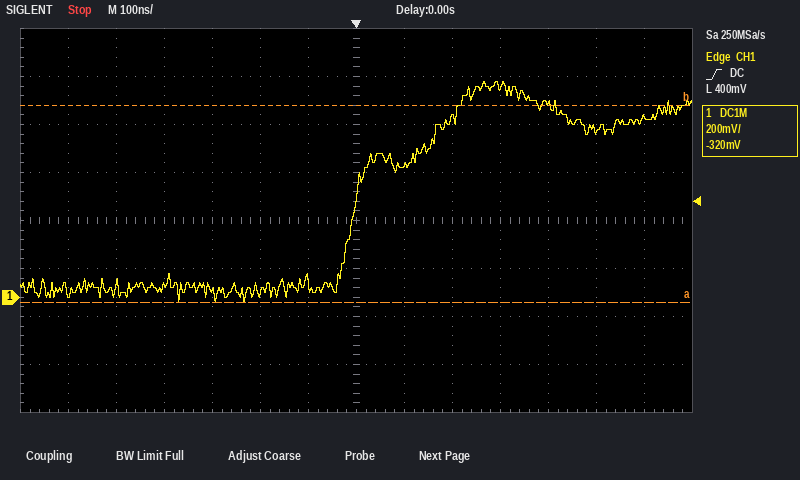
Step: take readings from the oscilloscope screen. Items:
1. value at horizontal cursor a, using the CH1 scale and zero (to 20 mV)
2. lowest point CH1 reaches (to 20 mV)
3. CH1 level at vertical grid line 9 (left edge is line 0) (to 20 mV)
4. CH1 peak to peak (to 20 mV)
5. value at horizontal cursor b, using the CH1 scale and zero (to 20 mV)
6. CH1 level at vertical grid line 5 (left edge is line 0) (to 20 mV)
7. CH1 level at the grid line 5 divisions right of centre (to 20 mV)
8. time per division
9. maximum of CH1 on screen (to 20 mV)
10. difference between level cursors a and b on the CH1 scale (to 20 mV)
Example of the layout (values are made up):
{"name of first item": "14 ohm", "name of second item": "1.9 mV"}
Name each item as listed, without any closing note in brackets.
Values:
{"value at horizontal cursor a, using the CH1 scale and zero": "-20 mV", "lowest point CH1 reaches": "-20 mV", "CH1 level at vertical grid line 9 (left edge is line 0)": "740 mV", "CH1 peak to peak": "920 mV", "value at horizontal cursor b, using the CH1 scale and zero": "800 mV", "CH1 level at vertical grid line 5 (left edge is line 0)": "20 mV", "CH1 level at the grid line 5 divisions right of centre": "700 mV", "time per division": "100 ns", "maximum of CH1 on screen": "900 mV", "difference between level cursors a and b on the CH1 scale": "820 mV"}
